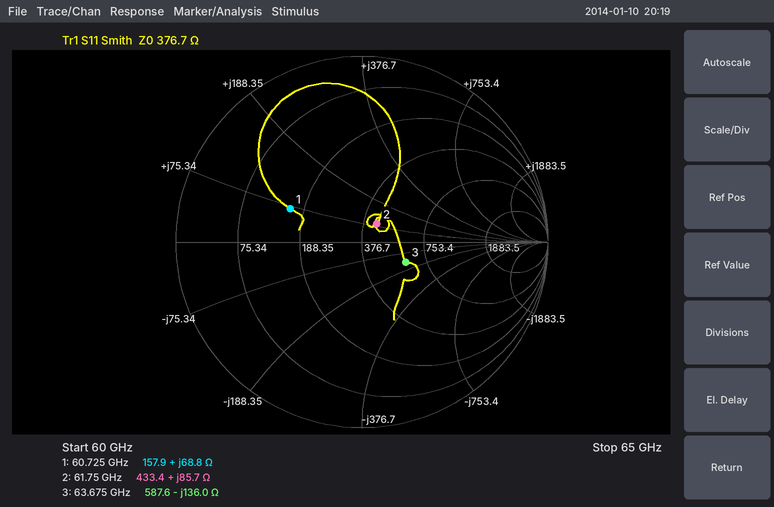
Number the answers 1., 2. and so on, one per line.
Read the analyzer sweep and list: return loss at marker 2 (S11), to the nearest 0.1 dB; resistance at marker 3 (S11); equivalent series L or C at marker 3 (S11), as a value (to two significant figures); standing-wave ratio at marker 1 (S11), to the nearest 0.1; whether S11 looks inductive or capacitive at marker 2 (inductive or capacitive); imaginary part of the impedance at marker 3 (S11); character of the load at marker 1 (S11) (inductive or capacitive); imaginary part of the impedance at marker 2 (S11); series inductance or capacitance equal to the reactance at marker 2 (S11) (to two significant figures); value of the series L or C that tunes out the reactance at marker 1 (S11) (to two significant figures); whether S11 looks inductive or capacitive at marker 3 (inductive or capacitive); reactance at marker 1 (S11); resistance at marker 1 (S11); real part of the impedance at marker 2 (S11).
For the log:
1. 18.0 dB
2. 587.6 Ω
3. 18 fF
4. 2.5
5. inductive
6. -136.0 Ω
7. inductive
8. +85.7 Ω
9. 220 pH
10. 38 fF
11. capacitive
12. +68.8 Ω
13. 157.9 Ω
14. 433.4 Ω
